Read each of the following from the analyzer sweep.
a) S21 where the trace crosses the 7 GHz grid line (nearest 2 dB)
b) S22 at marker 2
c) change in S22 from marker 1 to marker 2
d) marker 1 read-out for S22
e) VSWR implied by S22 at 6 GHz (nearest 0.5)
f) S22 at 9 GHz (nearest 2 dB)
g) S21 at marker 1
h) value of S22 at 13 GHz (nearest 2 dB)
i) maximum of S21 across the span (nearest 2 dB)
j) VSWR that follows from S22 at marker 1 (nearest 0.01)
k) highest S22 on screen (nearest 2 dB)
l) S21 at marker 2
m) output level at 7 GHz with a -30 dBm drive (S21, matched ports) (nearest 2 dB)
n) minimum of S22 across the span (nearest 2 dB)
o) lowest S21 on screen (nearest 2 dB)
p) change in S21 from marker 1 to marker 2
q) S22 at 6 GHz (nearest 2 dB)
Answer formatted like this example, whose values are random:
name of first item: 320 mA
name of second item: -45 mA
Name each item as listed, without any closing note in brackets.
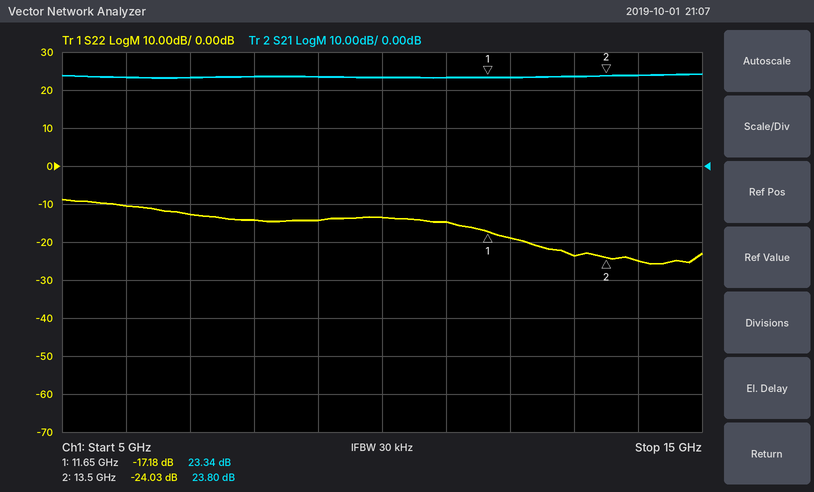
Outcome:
S21 where the trace crosses the 7 GHz grid line: 24 dB
S22 at marker 2: -24.03 dB
change in S22 from marker 1 to marker 2: -6.85 dB
marker 1 read-out for S22: -17.18 dB
VSWR implied by S22 at 6 GHz: 2.0
S22 at 9 GHz: -14 dB
S21 at marker 1: 23.34 dB
value of S22 at 13 GHz: -24 dB
maximum of S21 across the span: 24 dB
VSWR that follows from S22 at marker 1: 1.32
highest S22 on screen: -8 dB
S21 at marker 2: 23.80 dB
output level at 7 GHz with a -30 dBm drive (S21, matched ports): -6 dBm
minimum of S22 across the span: -26 dB
lowest S21 on screen: 24 dB
change in S21 from marker 1 to marker 2: 0.46 dB
S22 at 6 GHz: -10 dB
